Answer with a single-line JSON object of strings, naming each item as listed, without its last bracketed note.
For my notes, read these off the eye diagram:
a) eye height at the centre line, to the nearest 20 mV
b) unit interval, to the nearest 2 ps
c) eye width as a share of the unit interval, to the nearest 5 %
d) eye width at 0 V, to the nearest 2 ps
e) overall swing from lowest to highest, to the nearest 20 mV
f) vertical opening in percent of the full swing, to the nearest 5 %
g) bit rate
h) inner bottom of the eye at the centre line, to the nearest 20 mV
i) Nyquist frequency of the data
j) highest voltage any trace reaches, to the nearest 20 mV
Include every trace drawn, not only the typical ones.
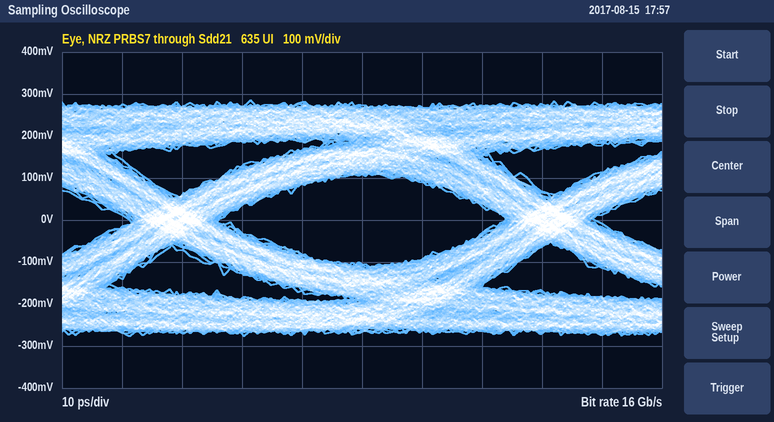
{"eye height at the centre line, to the nearest 20 mV": "220 mV", "unit interval, to the nearest 2 ps": "62 ps", "eye width as a share of the unit interval, to the nearest 5 %": "75 %", "eye width at 0 V, to the nearest 2 ps": "48 ps", "overall swing from lowest to highest, to the nearest 20 mV": "560 mV", "vertical opening in percent of the full swing, to the nearest 5 %": "40 %", "bit rate": "16 Gb/s", "inner bottom of the eye at the centre line, to the nearest 20 mV": "-100 mV", "Nyquist frequency of the data": "8 GHz", "highest voltage any trace reaches, to the nearest 20 mV": "280 mV"}
